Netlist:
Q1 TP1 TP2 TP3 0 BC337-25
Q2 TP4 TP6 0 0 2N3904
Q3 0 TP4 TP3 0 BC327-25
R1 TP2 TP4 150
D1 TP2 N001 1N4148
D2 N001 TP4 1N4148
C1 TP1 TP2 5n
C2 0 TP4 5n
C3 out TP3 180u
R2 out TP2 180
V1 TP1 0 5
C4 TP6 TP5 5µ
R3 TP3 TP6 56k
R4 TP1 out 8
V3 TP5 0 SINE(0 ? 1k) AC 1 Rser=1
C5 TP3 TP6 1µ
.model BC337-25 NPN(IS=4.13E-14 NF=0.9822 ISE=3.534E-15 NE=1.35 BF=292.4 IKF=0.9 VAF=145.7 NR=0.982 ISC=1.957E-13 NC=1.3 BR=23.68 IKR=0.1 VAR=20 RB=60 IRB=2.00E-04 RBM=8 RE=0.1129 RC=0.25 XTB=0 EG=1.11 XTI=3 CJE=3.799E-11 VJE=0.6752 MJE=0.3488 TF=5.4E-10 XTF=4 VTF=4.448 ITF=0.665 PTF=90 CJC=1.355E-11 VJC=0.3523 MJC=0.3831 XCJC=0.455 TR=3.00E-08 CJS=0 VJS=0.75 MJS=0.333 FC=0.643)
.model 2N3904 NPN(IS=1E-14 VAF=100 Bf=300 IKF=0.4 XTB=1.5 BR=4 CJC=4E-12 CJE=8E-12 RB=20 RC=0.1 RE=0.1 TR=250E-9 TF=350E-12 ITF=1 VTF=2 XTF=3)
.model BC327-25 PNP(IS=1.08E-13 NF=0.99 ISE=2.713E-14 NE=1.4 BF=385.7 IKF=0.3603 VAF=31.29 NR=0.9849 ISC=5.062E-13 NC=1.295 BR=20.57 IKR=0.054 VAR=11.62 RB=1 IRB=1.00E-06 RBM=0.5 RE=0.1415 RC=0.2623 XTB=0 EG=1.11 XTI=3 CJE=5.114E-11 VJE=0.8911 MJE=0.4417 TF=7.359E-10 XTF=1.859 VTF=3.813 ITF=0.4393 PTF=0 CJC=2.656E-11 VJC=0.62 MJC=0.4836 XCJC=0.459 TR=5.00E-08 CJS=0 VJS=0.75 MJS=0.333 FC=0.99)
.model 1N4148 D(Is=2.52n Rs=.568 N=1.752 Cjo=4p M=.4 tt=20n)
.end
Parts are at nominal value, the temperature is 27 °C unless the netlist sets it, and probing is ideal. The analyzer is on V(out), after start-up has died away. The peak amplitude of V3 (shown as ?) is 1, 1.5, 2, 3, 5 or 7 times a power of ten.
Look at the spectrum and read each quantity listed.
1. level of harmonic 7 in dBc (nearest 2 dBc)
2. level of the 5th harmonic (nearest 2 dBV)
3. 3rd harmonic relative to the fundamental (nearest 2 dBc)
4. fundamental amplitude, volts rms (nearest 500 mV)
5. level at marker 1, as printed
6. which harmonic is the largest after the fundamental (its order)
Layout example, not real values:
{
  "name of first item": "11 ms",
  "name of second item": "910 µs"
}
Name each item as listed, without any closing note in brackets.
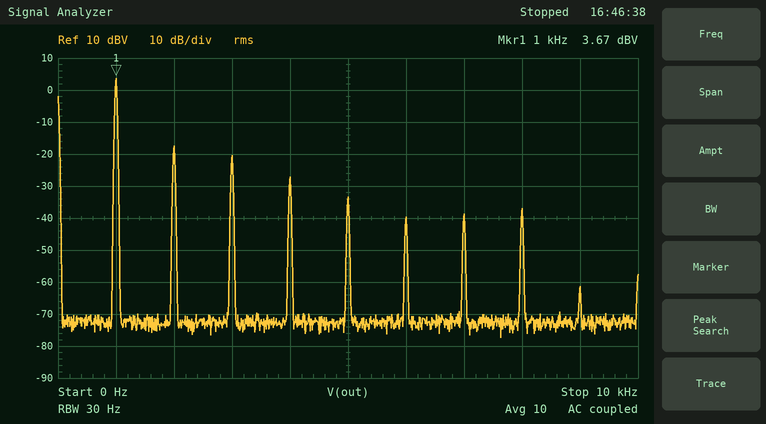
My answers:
{
  "level of harmonic 7 in dBc": "-42 dBc",
  "level of the 5th harmonic": "-34 dBV",
  "3rd harmonic relative to the fundamental": "-24 dBc",
  "fundamental amplitude, volts rms": "1.5 V",
  "level at marker 1, as printed": "3.67 dBV",
  "which harmonic is the largest after the fundamental": "2"
}
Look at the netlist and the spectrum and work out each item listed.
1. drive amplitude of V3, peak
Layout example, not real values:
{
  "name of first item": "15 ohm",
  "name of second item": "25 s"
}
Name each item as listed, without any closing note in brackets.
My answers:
{
  "drive amplitude of V3, peak": "500 mV"
}
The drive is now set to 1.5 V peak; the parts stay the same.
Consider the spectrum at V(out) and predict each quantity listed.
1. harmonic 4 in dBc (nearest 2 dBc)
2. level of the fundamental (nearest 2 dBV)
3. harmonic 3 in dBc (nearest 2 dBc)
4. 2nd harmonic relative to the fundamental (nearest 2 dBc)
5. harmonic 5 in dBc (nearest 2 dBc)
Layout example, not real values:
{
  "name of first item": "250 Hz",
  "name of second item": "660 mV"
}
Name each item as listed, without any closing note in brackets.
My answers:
{
  "harmonic 4 in dBc": "-40 dBc",
  "level of the fundamental": "2 dBV",
  "harmonic 3 in dBc": "-12 dBc",
  "2nd harmonic relative to the fundamental": "-4 dBc",
  "harmonic 5 in dBc": "-20 dBc"
}
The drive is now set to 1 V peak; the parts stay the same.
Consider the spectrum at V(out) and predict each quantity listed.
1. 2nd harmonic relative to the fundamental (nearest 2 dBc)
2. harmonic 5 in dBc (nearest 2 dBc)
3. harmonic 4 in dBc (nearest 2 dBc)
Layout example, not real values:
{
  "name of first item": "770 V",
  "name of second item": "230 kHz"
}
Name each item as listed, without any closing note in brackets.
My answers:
{
  "2nd harmonic relative to the fundamental": "-6 dBc",
  "harmonic 5 in dBc": "-28 dBc",
  "harmonic 4 in dBc": "-20 dBc"
}
